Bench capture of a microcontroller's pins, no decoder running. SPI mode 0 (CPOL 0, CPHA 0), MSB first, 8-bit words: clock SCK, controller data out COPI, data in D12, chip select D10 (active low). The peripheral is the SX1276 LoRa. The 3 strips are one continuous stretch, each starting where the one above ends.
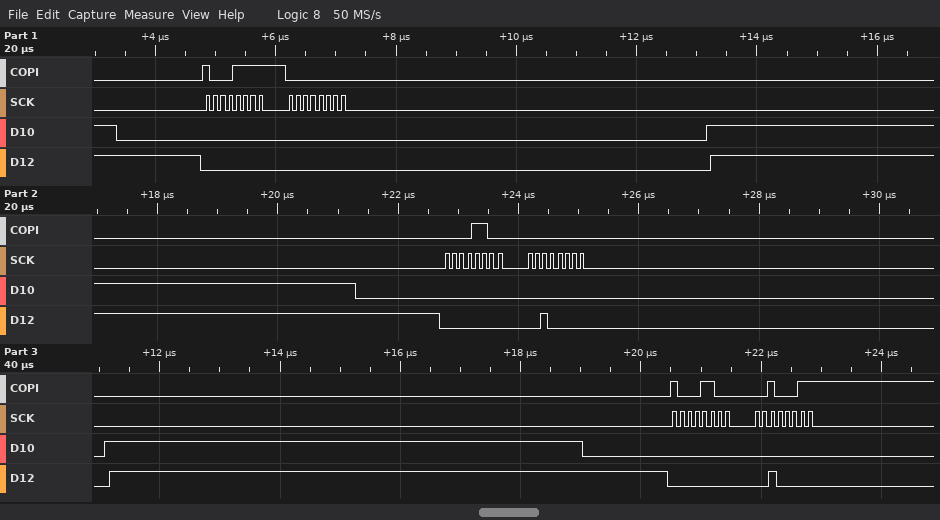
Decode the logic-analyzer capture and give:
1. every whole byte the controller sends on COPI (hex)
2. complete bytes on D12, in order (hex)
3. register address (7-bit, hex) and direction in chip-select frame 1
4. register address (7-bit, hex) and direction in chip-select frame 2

8F 00 0C 00 8C 23
00 00 00 20 00 20
0x0F write
0x0C read
